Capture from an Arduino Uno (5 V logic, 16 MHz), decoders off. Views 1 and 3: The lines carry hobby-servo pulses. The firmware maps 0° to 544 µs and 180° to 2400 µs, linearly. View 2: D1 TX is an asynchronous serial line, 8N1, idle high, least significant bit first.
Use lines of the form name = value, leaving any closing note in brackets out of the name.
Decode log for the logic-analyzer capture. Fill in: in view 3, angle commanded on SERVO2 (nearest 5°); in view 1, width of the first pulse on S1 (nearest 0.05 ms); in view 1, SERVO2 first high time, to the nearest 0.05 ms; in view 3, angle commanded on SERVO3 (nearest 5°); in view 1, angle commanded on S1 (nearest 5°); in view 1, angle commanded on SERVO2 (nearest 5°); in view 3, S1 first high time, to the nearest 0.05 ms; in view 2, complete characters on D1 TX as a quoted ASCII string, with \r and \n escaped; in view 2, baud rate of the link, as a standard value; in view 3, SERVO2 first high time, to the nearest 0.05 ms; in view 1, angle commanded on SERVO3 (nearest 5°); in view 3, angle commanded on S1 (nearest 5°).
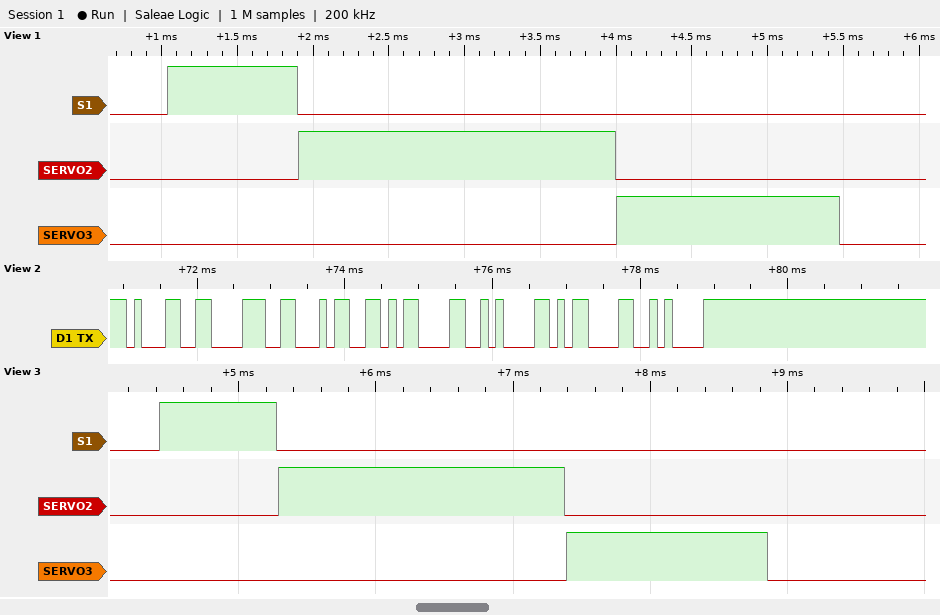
in view 3, angle commanded on SERVO2 = 150°
in view 1, width of the first pulse on S1 = 0.85 ms
in view 1, SERVO2 first high time, to the nearest 0.05 ms = 2.10 ms
in view 3, angle commanded on SERVO3 = 90°
in view 1, angle commanded on S1 = 30°
in view 1, angle commanded on SERVO2 = 150°
in view 3, S1 first high time, to the nearest 0.05 ms = 0.85 ms
in view 2, complete characters on D1 TX as a quoted ASCII string, with \r and \n escaped = "184\r\n\r\n"
in view 2, baud rate of the link, as a standard value = 9600 baud
in view 3, SERVO2 first high time, to the nearest 0.05 ms = 2.10 ms
in view 1, angle commanded on SERVO3 = 90°
in view 3, angle commanded on S1 = 30°
